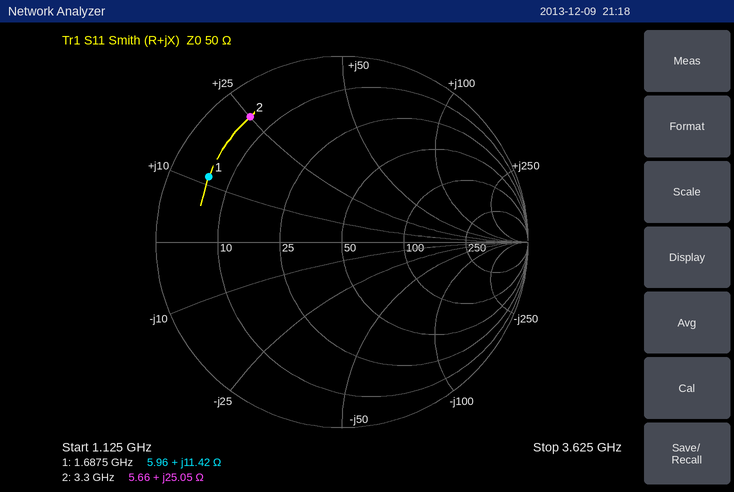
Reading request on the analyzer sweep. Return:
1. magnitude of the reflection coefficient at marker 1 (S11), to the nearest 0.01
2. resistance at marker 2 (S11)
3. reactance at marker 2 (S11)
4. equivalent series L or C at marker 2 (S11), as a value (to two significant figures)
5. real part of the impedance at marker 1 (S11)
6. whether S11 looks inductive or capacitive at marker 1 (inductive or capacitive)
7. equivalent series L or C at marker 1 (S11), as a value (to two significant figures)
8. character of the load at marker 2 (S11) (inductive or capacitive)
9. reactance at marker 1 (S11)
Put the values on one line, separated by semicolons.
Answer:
0.80; 5.66 Ω; +25.05 Ω; 1.2 nH; 5.96 Ω; inductive; 1.1 nH; inductive; +11.42 Ω
